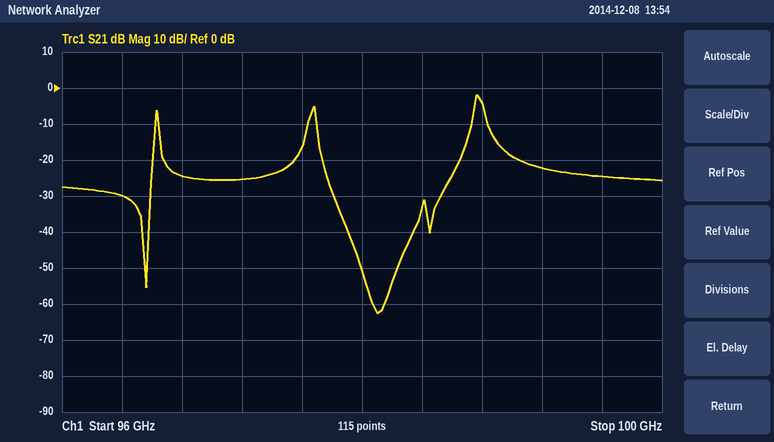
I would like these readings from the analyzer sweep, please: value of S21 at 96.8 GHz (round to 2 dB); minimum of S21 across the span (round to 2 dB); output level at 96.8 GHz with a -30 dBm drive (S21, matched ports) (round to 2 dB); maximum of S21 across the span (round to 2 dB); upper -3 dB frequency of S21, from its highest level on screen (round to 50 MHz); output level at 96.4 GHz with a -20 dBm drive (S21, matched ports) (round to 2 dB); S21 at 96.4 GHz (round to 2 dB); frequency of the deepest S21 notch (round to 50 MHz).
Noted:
-24 dB
-62 dB
-54 dBm
-2 dB
98.80 GHz
-50 dBm
-30 dB
98.10 GHz
